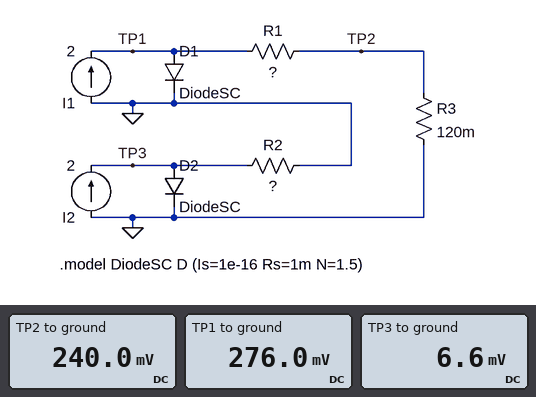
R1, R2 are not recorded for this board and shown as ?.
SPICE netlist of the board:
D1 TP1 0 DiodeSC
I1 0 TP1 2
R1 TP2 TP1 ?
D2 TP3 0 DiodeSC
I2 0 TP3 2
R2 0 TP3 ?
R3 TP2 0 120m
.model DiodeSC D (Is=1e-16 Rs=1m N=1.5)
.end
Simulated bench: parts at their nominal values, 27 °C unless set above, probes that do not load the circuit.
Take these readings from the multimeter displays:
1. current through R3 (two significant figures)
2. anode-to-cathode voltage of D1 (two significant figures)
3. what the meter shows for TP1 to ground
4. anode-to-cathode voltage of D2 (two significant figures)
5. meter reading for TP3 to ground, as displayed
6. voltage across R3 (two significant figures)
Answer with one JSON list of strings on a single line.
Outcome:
["2.0 A", "280 mV", "276.0 mV", "6.6 mV", "6.6 mV", "240 mV"]
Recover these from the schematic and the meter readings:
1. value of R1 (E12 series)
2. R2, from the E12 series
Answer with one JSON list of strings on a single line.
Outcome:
["0.018 Ω", "3.3 mΩ"]
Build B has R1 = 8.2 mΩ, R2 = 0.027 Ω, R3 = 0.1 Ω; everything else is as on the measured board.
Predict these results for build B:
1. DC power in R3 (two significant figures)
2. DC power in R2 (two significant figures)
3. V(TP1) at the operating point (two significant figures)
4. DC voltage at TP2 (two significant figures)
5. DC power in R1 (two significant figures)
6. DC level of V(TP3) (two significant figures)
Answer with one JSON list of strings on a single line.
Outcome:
["400 mW", "110 mW", "220 mV", "200 mV", "33 mW", "54 mV"]
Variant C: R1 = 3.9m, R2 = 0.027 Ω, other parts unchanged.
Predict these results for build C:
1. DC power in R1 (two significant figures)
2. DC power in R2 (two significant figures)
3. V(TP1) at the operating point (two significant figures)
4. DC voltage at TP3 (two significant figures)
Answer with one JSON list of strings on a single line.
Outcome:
["16 mW", "110 mW", "250 mV", "54 mV"]
